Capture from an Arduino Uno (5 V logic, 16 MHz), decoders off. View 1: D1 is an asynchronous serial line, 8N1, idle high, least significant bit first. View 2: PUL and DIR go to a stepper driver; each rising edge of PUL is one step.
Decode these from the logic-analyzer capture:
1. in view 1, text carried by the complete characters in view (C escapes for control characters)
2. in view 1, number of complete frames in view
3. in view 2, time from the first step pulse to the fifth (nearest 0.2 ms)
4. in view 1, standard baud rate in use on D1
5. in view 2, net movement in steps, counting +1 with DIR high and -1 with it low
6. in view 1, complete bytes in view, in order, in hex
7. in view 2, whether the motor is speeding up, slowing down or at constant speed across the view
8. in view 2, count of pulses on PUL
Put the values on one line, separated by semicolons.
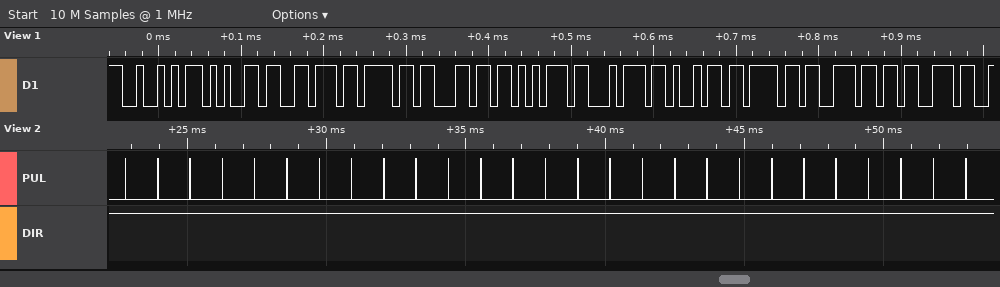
"Revolutions"; 11; 4.6 ms; 115200 baud; +27; 52 65 76 6F 6C 75 74 69 6F 6E 73; constant speed; 27
